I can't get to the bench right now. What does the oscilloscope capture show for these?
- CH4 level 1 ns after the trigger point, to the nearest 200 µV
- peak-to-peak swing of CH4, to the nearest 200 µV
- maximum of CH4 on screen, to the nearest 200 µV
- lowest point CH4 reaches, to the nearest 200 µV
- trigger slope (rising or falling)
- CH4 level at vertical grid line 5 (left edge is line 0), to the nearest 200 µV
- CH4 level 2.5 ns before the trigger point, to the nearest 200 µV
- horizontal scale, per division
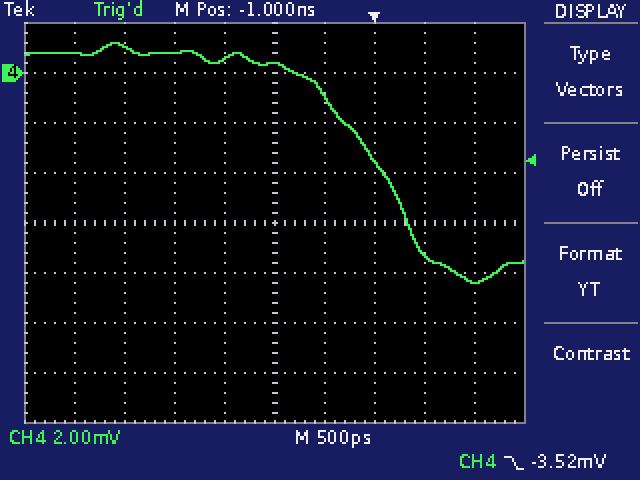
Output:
-8.4 mV
9.6 mV
1.2 mV
-8.4 mV
falling
400 µV
1.0 mV
500 ps
